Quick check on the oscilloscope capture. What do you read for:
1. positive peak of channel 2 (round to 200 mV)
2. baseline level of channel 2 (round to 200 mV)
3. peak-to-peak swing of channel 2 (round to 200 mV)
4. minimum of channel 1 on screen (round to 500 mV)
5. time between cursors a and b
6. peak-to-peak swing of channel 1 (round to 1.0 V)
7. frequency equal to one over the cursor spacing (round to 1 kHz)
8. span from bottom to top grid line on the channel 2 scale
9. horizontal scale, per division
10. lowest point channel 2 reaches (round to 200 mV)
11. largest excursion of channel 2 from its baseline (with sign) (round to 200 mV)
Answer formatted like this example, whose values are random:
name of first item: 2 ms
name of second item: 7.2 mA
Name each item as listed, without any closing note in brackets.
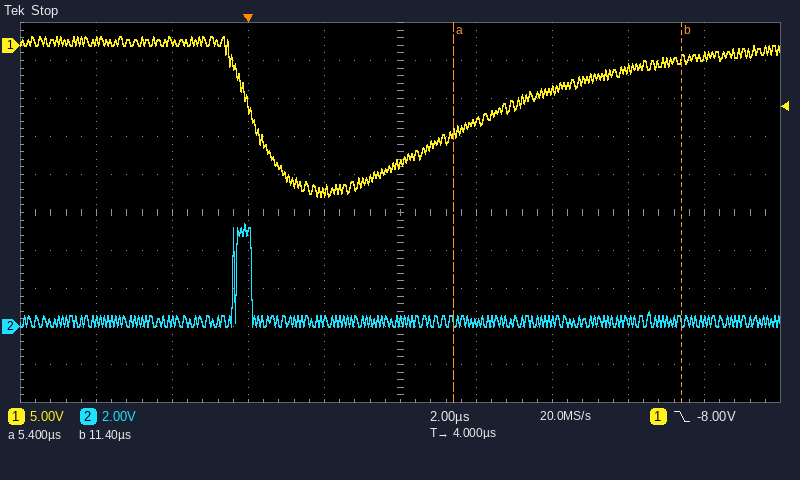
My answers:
positive peak of channel 2: 5.4 V
baseline level of channel 2: 200 mV
peak-to-peak swing of channel 2: 5.4 V
minimum of channel 1 on screen: -20.0 V
time between cursors a and b: 6.0 µs
peak-to-peak swing of channel 1: 21.0 V
frequency equal to one over the cursor spacing: 167 kHz
span from bottom to top grid line on the channel 2 scale: 20 V
horizontal scale, per division: 2 µs
lowest point channel 2 reaches: 0.0 V
largest excursion of channel 2 from its baseline (with sign): +5.2 V
